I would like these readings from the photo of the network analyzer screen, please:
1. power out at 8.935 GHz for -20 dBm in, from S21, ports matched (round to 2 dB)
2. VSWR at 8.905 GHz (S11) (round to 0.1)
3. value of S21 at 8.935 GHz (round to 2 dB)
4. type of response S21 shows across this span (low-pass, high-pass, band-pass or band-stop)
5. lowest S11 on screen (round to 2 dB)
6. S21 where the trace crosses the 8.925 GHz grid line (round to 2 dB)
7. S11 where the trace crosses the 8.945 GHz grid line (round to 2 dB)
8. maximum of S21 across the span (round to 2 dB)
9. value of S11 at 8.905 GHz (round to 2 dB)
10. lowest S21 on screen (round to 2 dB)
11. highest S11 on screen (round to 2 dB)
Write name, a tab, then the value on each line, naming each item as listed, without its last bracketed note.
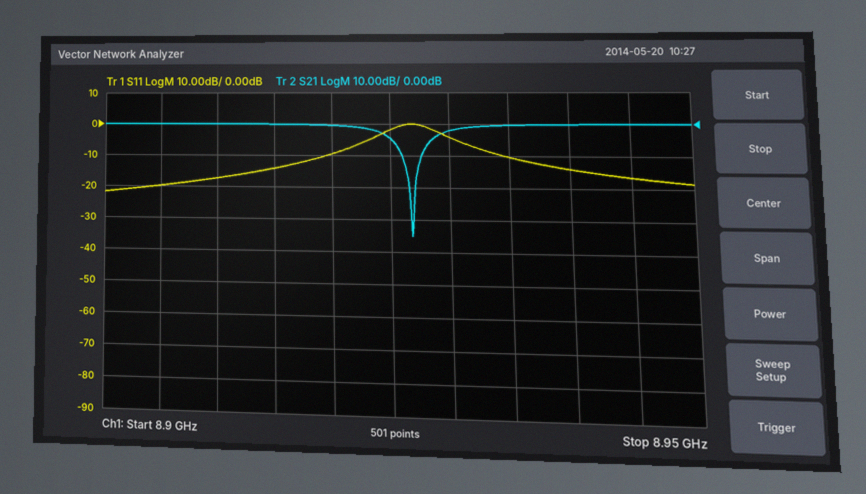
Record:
power out at 8.935 GHz for -20 dBm in, from S21, ports matched	-20 dBm
VSWR at 8.905 GHz (S11)	1.2
value of S21 at 8.935 GHz	0 dB
type of response S21 shows across this span	band-stop
lowest S11 on screen	-22 dB
S21 where the trace crosses the 8.925 GHz grid line	-4 dB
S11 where the trace crosses the 8.945 GHz grid line	-16 dB
maximum of S21 across the span	0 dB
value of S11 at 8.905 GHz	-20 dB
lowest S21 on screen	-36 dB
highest S11 on screen	0 dB
